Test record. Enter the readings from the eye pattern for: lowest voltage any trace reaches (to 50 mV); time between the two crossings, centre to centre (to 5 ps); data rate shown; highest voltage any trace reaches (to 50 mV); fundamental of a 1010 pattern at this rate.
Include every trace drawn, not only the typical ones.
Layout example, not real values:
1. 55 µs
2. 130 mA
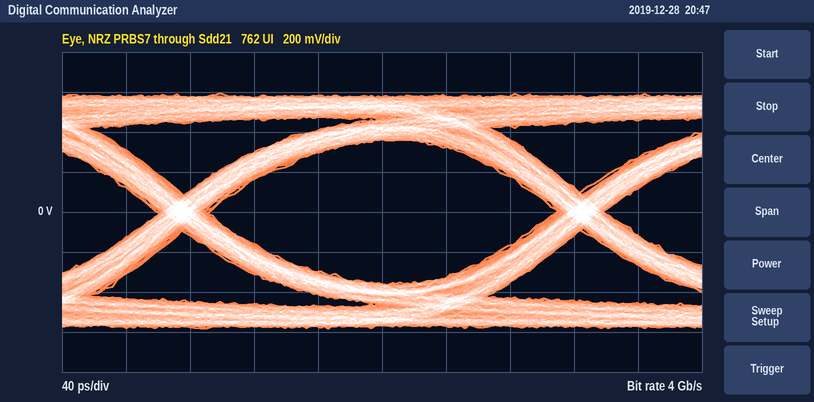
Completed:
1. -600 mV
2. 250 ps
3. 4 Gb/s
4. 600 mV
5. 2 GHz
